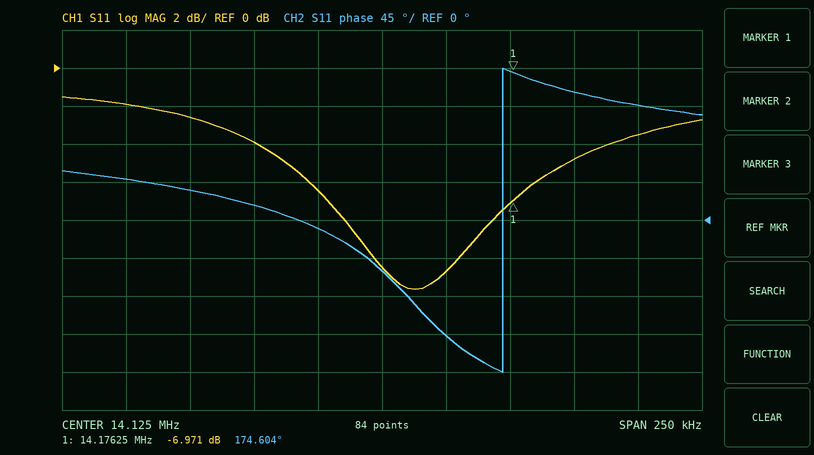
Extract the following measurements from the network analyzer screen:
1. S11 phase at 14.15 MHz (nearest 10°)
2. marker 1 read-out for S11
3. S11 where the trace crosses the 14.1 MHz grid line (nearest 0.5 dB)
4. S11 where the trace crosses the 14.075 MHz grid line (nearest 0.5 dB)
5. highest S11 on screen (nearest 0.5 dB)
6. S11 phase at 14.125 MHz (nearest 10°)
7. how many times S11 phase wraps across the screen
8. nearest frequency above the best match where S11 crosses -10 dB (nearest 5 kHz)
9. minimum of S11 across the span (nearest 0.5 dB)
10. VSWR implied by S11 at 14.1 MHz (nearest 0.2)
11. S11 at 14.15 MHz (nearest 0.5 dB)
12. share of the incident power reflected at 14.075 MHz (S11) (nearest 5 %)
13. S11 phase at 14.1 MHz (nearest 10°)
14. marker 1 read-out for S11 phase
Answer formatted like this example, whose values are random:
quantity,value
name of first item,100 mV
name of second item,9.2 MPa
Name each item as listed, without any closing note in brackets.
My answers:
quantity,value
S11 phase at 14.15 MHz,-140°
marker 1 read-out for S11,-6.971 dB
S11 where the trace crosses the 14.1 MHz grid line,-6.5 dB
S11 where the trace crosses the 14.075 MHz grid line,-4.0 dB
highest S11 on screen,-1.5 dB
S11 phase at 14.125 MHz,-60°
how many times S11 phase wraps across the screen,1
nearest frequency above the best match where S11 crosses -10 dB,14.155 MHz
minimum of S11 across the span,-11.5 dB
VSWR implied by S11 at 14.1 MHz,2.8
S11 at 14.15 MHz,-10.5 dB
share of the incident power reflected at 14.075 MHz (S11),40 %
S11 phase at 14.1 MHz,-10°
marker 1 read-out for S11 phase,174.604°
